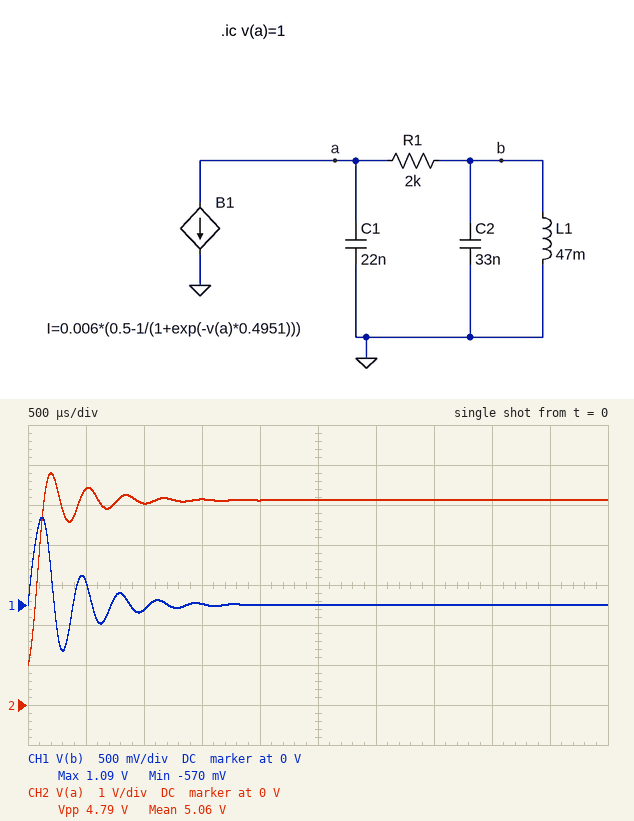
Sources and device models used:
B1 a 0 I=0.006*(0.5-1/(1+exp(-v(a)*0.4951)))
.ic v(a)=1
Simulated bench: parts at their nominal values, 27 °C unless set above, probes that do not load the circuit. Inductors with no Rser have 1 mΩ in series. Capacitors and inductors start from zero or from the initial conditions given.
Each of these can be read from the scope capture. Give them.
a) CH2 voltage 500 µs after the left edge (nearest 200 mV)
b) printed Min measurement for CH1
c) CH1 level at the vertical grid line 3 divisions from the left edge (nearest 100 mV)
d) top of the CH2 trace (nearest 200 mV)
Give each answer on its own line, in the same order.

5.4 V
-570 mV
0 V
5.8 V
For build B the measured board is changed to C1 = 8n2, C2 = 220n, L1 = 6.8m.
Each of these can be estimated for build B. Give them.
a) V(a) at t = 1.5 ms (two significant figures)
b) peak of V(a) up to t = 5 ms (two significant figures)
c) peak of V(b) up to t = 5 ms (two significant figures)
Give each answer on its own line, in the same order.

4.6 V
5.9 V
640 mV
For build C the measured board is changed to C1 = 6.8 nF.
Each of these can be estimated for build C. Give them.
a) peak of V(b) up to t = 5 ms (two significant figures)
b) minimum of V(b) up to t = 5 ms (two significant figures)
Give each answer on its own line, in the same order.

59 V
-59 V
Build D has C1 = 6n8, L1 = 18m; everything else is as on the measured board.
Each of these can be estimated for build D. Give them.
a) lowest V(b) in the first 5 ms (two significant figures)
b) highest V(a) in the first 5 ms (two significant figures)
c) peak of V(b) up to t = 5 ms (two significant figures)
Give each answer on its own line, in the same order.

-1.7 V
7.1 V
1.8 V
